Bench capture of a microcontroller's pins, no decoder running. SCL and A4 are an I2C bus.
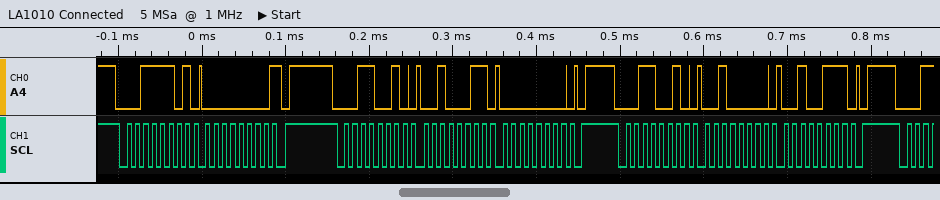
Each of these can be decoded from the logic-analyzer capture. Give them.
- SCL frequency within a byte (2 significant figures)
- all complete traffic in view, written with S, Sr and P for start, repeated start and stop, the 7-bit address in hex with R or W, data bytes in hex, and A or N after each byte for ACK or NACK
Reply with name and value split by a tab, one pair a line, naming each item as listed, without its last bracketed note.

SCL frequency within a byte	100 kHz
all complete traffic in view, written with S, Sr and P for start, repeated start and stop, the 7-bit address in hex with R or W, data bytes in hex, and A or N after each byte for ACK or NACK	S 1ER A 00 N P S 19W A 23 A 00 A P S 19W A 20 A 27 A P
